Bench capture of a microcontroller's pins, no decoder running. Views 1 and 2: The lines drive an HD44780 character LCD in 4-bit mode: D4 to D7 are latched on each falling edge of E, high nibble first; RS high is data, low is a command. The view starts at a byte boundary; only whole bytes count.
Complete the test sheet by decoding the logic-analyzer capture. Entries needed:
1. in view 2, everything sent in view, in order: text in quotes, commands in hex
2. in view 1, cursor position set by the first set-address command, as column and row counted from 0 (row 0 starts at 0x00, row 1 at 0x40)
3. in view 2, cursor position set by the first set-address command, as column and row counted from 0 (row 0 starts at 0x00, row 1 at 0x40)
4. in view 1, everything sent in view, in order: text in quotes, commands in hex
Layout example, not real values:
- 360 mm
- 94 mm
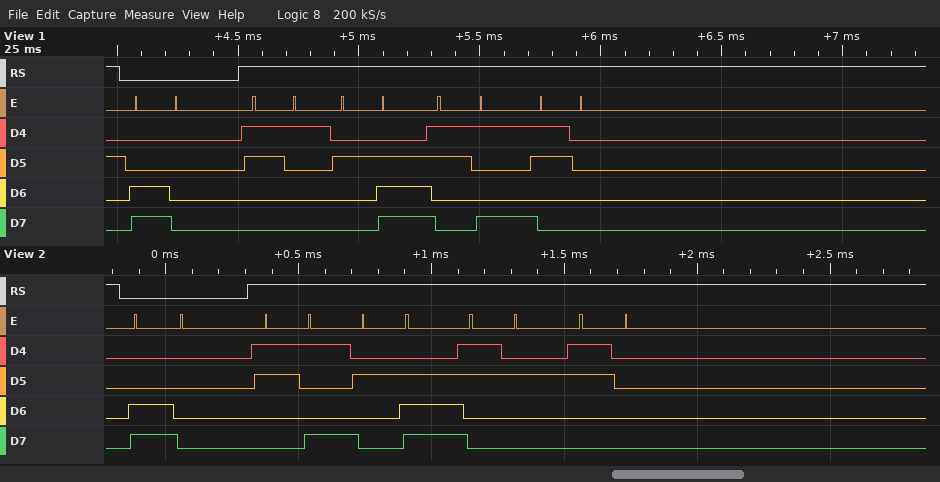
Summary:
- 0xC0 "9.20"
- column 0, row 1
- column 0, row 1
- 0xC0 "1.90"
